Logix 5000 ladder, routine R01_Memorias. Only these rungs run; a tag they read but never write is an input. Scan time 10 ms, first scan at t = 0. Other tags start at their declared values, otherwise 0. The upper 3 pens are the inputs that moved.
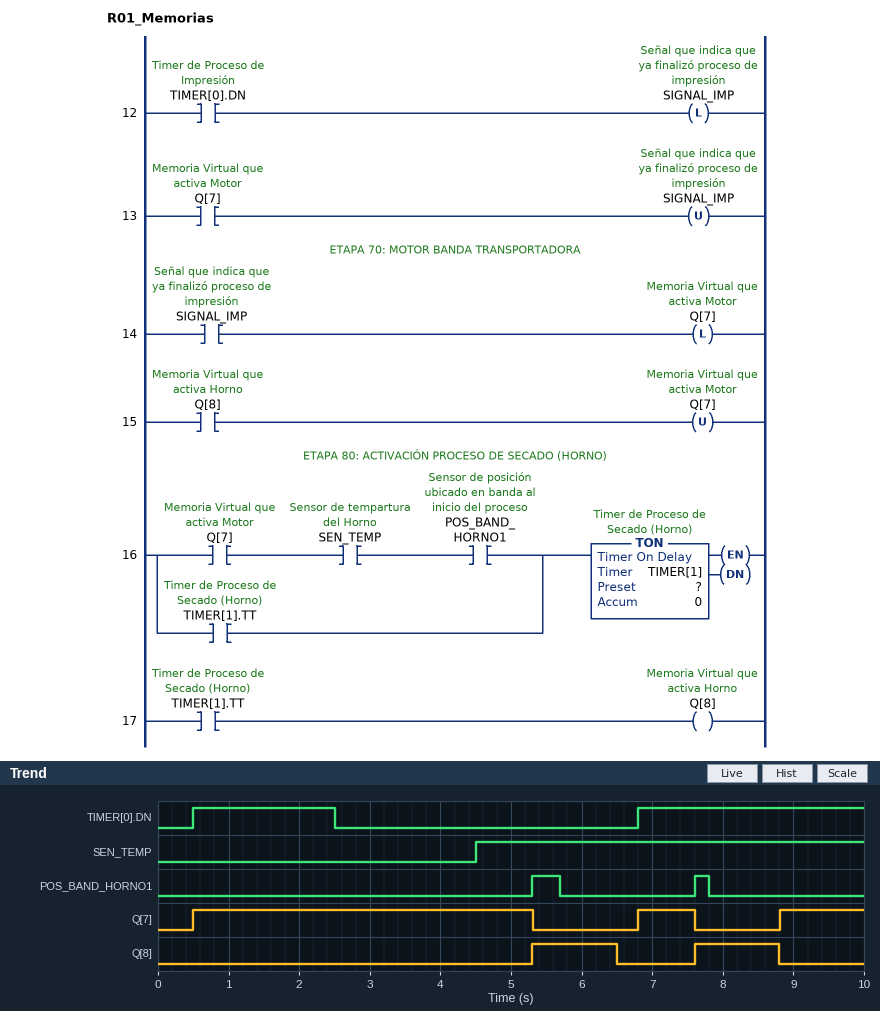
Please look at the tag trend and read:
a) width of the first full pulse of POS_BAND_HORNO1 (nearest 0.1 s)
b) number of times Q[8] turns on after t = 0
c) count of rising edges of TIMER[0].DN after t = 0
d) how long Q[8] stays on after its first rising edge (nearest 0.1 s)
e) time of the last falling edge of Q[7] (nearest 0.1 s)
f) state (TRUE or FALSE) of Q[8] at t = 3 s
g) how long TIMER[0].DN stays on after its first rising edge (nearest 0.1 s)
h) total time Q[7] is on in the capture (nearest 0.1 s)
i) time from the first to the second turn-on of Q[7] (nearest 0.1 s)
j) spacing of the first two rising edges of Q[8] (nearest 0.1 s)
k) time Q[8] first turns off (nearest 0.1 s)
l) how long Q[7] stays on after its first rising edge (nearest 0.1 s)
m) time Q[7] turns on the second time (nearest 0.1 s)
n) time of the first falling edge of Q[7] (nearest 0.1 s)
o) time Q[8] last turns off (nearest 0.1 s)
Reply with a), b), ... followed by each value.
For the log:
a) 0.4 s
b) 2
c) 2
d) 1.2 s
e) 7.6 s
f) FALSE
g) 2.0 s
h) 6.8 s
i) 6.3 s
j) 2.3 s
k) 6.5 s
l) 4.8 s
m) 6.8 s
n) 5.3 s
o) 8.8 s
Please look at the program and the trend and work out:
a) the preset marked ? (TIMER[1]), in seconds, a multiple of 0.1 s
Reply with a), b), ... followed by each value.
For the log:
a) 1.2 s
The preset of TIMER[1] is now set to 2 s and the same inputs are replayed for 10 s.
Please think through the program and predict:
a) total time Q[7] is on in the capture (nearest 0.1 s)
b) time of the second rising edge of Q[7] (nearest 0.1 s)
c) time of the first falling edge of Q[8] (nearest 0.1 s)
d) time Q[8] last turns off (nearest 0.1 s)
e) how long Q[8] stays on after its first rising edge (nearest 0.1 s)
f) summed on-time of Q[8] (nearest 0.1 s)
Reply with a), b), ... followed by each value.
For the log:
a) 5.5 s
b) 7.3 s
c) 7.3 s
d) 9.6 s
e) 2.0 s
f) 4.0 s
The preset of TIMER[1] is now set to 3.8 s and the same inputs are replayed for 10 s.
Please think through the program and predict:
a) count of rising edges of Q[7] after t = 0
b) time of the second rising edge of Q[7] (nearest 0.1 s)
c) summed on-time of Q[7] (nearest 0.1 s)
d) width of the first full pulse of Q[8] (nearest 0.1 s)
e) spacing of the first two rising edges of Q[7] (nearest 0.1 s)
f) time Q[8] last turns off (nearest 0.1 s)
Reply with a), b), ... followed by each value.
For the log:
a) 2
b) 9.1 s
c) 5.7 s
d) 3.8 s
e) 8.6 s
f) 9.1 s
